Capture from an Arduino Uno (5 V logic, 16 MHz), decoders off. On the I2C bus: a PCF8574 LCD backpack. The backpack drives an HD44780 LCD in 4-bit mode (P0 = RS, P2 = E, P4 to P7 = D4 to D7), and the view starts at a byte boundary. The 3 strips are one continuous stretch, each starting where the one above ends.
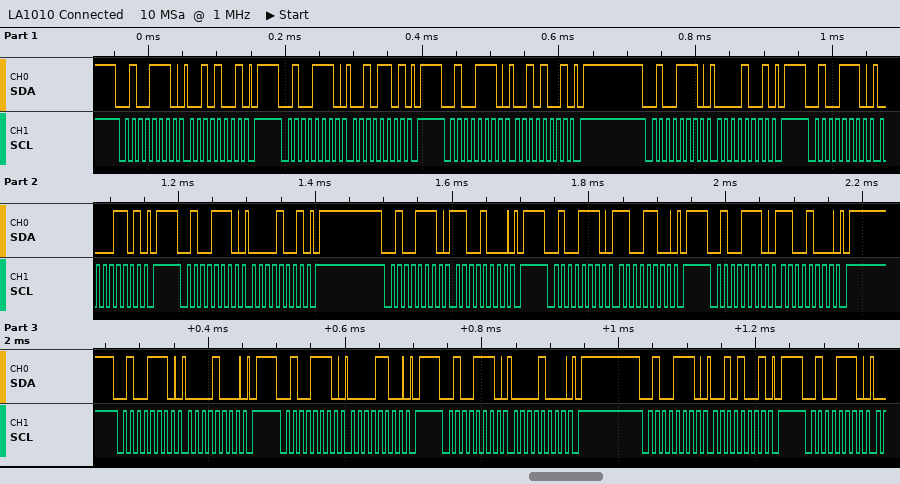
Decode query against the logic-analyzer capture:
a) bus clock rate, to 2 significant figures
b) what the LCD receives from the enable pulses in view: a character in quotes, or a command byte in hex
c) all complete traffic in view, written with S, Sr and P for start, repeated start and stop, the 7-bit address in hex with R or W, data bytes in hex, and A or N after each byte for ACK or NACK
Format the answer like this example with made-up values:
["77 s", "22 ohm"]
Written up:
["100 kHz", "' ' 0xC0", "S 27W A 29 A P S 27W A 2D A P S 27W A 29 A P S 27W A 09 A P S 27W A 0D A P S 27W A 09 A P S 27W A C8 A P S 27W A CC A P S 27W A C8 A P S 27W A 08 A P S 27W A 0C A P S 27W A 08 A P S 27W A 29 A P S 27W A"]
